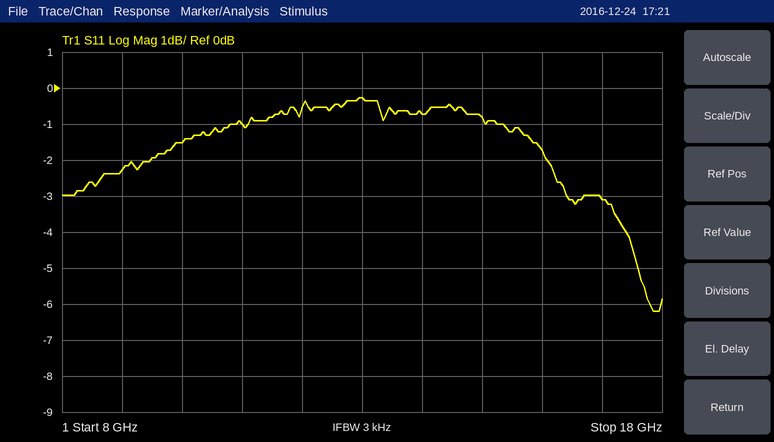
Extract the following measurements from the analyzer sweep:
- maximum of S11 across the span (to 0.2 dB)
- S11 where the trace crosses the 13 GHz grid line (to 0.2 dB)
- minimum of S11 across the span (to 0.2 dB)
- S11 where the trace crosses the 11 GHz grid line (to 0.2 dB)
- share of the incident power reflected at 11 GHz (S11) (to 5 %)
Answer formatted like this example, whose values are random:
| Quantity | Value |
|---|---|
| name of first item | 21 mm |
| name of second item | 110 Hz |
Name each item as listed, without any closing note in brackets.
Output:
| Quantity | Value |
|---|---|
| maximum of S11 across the span | -0.2 dB |
| S11 where the trace crosses the 13 GHz grid line | -0.2 dB |
| minimum of S11 across the span | -6.2 dB |
| S11 where the trace crosses the 11 GHz grid line | -1.0 dB |
| share of the incident power reflected at 11 GHz (S11) | 80 % |
